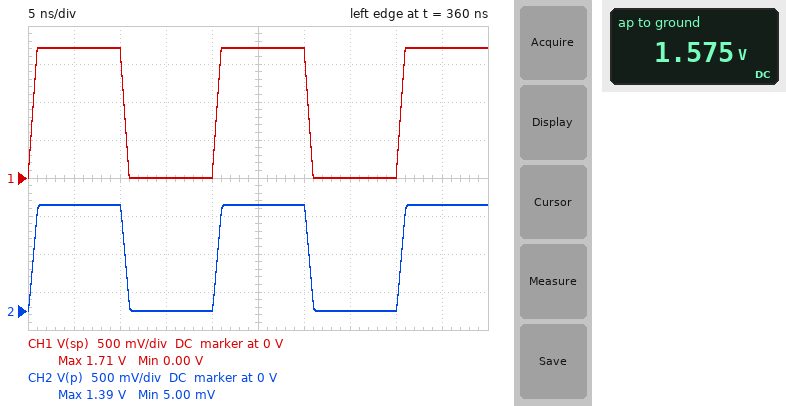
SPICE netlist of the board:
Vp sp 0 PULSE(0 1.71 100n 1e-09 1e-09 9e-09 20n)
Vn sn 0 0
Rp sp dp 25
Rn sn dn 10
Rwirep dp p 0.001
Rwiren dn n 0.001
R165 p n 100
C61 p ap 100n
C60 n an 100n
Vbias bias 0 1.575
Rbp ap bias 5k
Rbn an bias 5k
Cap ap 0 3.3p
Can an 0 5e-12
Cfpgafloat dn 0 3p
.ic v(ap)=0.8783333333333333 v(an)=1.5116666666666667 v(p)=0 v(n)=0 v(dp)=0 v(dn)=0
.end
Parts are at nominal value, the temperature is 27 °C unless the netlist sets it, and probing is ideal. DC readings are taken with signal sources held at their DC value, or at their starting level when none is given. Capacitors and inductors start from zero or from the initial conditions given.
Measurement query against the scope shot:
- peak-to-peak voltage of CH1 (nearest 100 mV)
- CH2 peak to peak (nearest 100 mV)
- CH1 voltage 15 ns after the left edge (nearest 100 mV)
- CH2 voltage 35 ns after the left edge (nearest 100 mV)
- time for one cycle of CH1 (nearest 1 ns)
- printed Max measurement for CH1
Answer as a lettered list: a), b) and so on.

a) 1.7 V
b) 1.4 V
c) 0 V
d) 0 V
e) 20 ns
f) 1.71 V
